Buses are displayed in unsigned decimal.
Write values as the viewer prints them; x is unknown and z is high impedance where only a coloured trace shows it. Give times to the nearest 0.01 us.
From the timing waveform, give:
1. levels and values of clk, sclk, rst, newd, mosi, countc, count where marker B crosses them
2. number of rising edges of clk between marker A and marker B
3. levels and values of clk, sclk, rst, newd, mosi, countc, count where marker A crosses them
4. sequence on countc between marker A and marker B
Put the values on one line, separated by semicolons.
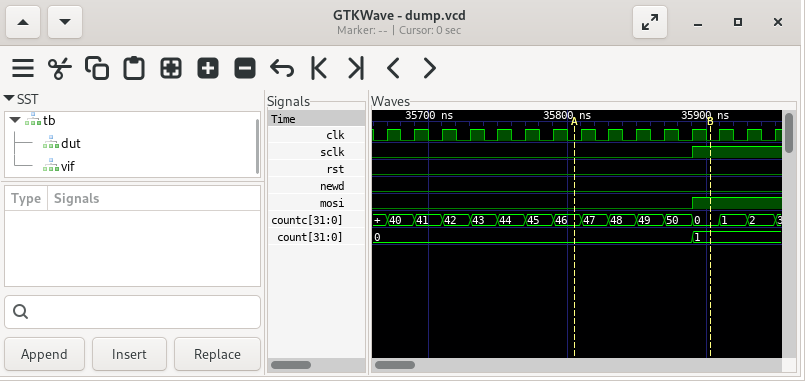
clk=0, sclk=1, rst=0, newd=0, mosi=1, countc=0, count=1; 5; clk=0, sclk=0, rst=0, newd=0, mosi=0, countc=46, count=0; 46, 47, 48, 49, 50, 0
